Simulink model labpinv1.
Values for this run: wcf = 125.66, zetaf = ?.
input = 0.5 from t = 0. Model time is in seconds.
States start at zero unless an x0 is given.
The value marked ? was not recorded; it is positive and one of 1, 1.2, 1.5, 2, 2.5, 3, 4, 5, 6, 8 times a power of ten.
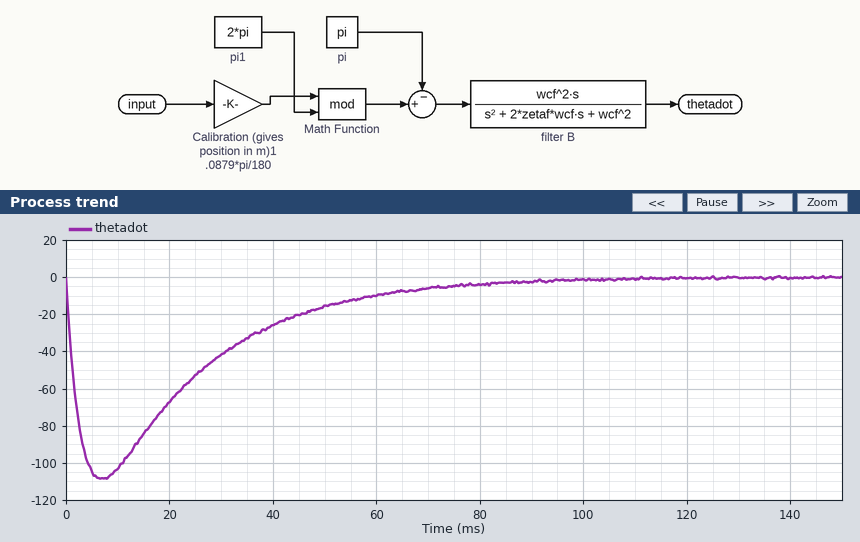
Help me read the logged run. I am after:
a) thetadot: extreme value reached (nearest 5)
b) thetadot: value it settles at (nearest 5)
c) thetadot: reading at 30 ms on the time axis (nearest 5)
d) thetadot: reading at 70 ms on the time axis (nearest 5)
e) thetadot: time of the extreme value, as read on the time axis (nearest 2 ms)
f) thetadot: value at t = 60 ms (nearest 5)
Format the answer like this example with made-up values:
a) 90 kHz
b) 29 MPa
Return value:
a) -110
b) 0
c) -40
d) -5
e) 6 ms
f) -10
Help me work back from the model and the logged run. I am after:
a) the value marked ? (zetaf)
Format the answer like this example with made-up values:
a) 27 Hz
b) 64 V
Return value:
a) 1.5
